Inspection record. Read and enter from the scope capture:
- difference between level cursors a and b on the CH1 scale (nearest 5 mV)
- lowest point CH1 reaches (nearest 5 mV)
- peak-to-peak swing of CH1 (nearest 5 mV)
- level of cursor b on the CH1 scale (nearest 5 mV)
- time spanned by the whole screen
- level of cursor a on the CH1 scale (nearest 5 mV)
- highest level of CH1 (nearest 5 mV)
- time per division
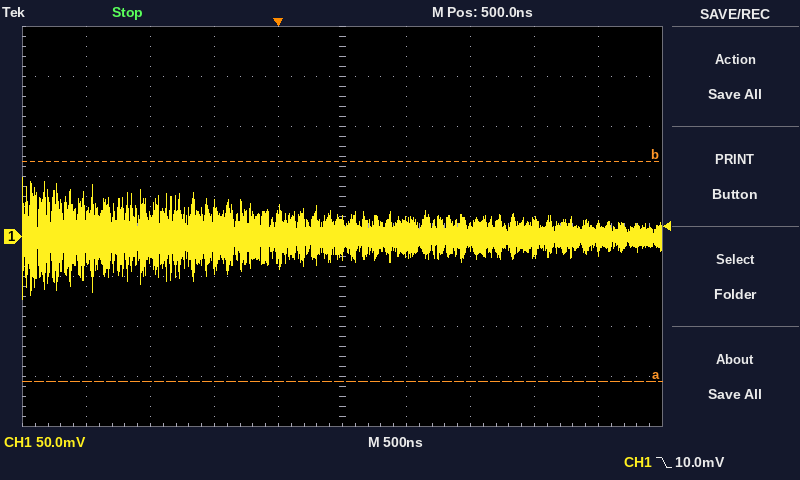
220 mV
-60 mV
120 mV
75 mV
5 µs
-145 mV
60 mV
500 ns
